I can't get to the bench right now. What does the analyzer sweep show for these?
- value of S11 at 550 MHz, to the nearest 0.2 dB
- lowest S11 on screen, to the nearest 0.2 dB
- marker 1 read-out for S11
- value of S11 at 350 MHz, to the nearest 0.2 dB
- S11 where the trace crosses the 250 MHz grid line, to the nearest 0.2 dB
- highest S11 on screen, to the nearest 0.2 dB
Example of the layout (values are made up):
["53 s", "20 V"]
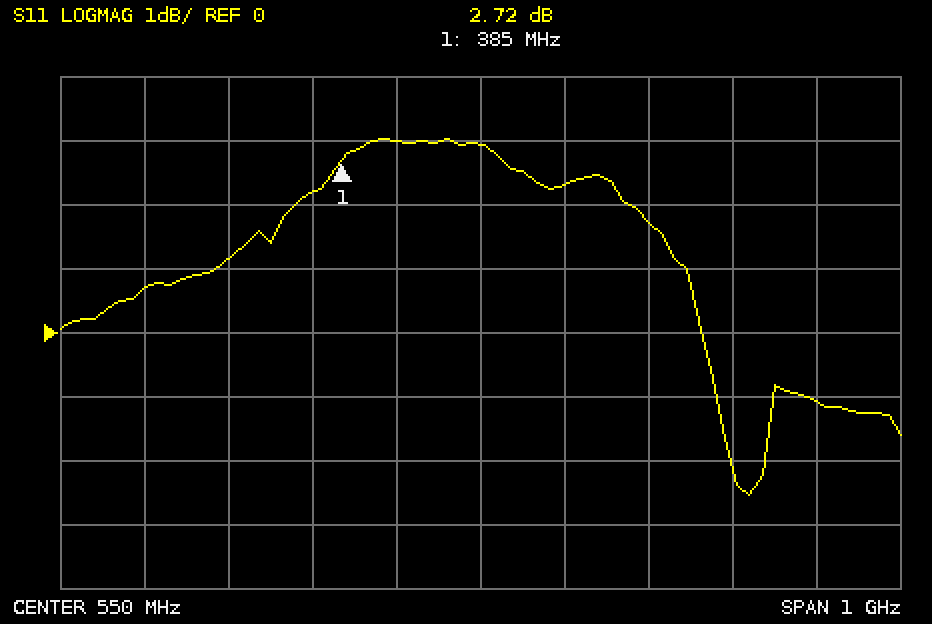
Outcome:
["3.0 dB", "-2.6 dB", "2.72 dB", "2.2 dB", "1.2 dB", "3.0 dB"]
